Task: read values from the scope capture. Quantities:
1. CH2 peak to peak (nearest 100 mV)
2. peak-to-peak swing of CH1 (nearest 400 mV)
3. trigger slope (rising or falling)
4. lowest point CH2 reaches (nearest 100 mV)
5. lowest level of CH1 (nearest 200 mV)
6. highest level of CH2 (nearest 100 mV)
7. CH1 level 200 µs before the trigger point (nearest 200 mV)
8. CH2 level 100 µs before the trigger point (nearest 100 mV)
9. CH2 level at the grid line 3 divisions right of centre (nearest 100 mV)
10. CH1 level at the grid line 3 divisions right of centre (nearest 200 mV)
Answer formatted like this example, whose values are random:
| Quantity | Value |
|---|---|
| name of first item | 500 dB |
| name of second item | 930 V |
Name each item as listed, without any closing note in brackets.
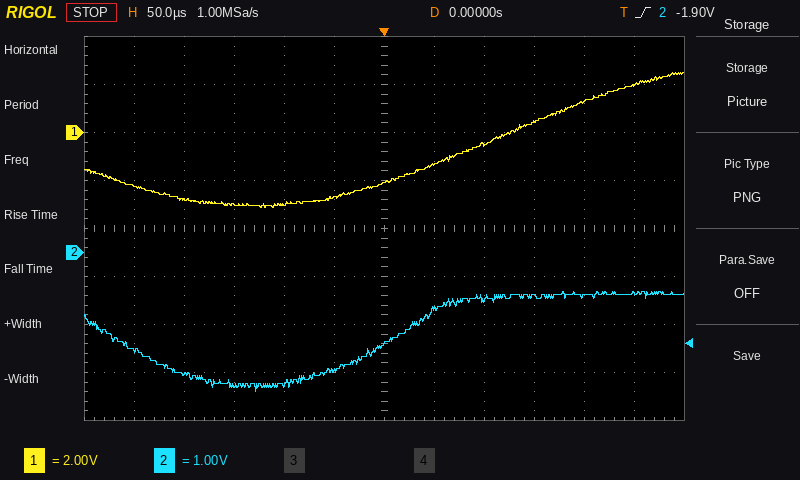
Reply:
| Quantity | Value |
|---|---|
| CH2 peak to peak | 2.1 V |
| peak-to-peak swing of CH1 | 5.6 V |
| trigger slope | rising |
| lowest point CH2 reaches | -2.9 V |
| lowest level of CH1 | -3.2 V |
| highest level of CH2 | -800 mV |
| CH1 level 200 µs before the trigger point | -2.8 V |
| CH2 level 100 µs before the trigger point | -2.7 V |
| CH2 level at the grid line 3 divisions right of centre | -900 mV |
| CH1 level at the grid line 3 divisions right of centre | 400 mV |
